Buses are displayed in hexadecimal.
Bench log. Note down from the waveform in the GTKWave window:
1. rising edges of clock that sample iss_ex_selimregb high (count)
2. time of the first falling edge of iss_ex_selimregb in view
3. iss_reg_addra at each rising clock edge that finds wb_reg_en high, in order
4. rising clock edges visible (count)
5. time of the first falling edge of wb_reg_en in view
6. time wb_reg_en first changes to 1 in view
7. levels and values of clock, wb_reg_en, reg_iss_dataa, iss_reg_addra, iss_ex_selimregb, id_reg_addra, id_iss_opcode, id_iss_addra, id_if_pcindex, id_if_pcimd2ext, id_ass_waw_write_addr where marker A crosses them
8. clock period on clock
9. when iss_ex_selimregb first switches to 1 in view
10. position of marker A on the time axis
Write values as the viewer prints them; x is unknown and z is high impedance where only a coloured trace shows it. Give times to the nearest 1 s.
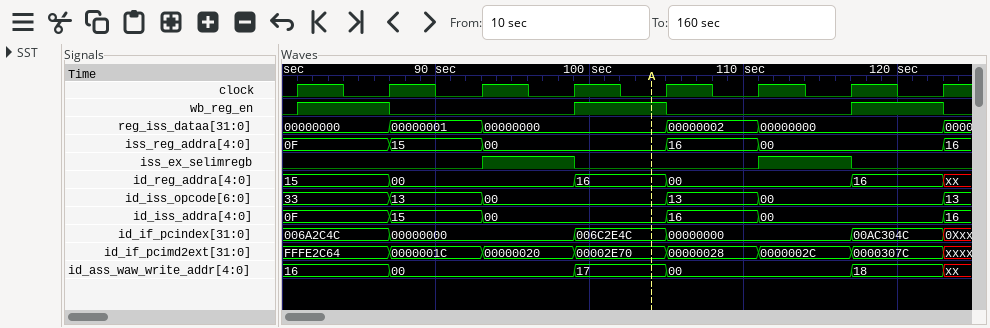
2
99 s
0F, 00, 00
8
87 s
81 s
clock=0, wb_reg_en=1, reg_iss_dataa=00000000, iss_reg_addra=00, iss_ex_selimregb=0, id_reg_addra=16, id_iss_opcode=00, id_iss_addra=00, id_if_pcindex=006C2E4C, id_if_pcimd2ext=00002E70, id_ass_waw_write_addr=17
6 s
93 s
104 s
